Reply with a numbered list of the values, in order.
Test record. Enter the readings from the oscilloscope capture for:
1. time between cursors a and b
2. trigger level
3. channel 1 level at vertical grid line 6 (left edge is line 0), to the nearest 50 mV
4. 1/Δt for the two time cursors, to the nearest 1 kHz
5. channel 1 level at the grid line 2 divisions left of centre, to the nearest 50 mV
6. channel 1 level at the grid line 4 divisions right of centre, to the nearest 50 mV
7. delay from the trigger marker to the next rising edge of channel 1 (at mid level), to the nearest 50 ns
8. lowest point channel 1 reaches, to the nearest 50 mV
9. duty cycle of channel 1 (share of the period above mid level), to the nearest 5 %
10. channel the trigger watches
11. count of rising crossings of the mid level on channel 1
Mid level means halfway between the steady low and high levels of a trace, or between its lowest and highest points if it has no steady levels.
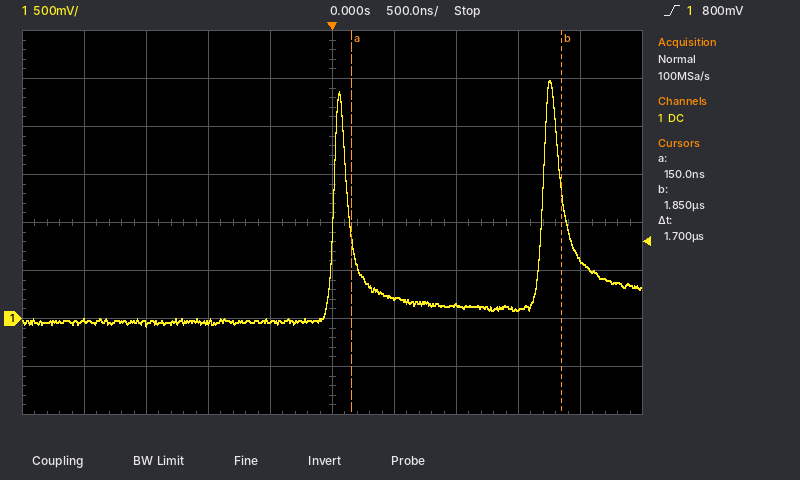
1. 1.7 µs
2. 800 mV
3. 200 mV
4. 588 kHz
5. -50 mV
6. 600 mV
7. 1.70 µs
8. -100 mV
9. 10 %
10. channel 1
11. 2
